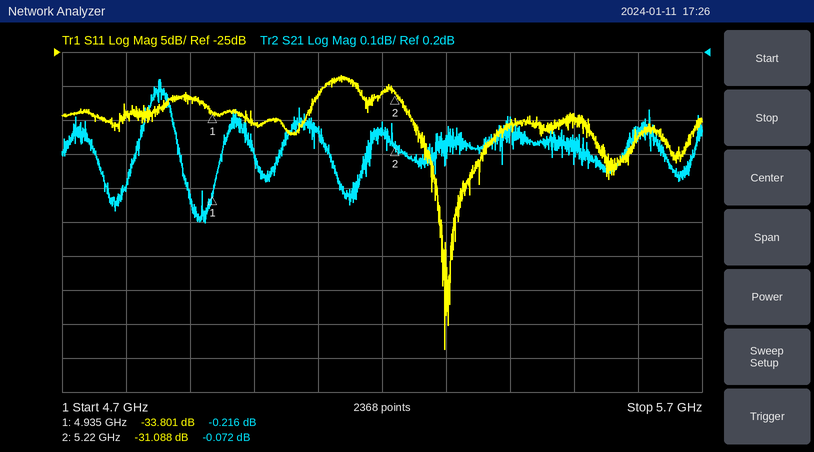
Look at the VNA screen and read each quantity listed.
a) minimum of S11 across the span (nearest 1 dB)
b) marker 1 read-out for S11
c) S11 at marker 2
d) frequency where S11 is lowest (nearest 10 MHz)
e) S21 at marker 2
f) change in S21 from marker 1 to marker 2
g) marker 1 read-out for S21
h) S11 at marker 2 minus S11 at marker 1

-69 dB
-33.801 dB
-31.088 dB
5.30 GHz
-0.072 dB
0.144 dB
-0.216 dB
2.713 dB
